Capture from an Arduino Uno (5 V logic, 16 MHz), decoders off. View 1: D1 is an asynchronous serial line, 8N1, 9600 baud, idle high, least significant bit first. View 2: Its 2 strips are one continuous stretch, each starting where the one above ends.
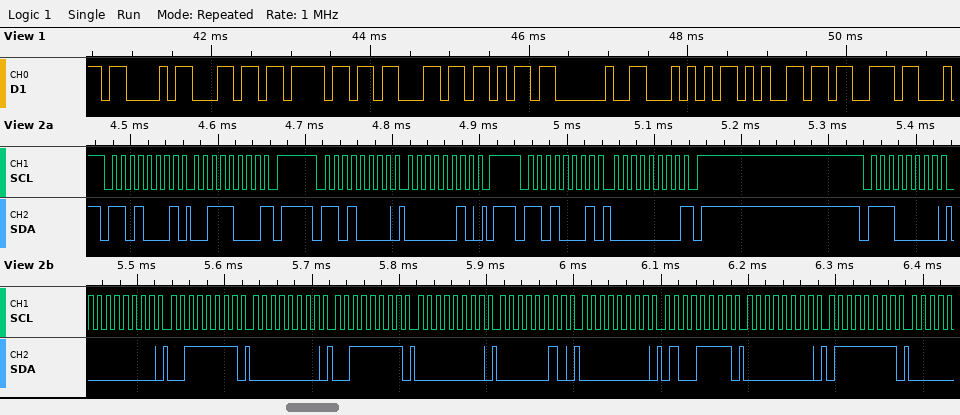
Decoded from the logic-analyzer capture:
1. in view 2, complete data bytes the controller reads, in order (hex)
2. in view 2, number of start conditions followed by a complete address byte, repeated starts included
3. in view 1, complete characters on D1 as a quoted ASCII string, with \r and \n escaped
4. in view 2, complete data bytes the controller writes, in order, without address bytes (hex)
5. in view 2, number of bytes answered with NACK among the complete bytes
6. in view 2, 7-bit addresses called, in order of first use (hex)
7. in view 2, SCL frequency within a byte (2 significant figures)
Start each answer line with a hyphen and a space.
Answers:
- 38 00
- 4
- "Clock Tes"
- 02 00 3F 00 3F 00 02 00 4F 00 7F
- 2
- 0x68 0x70
- 100 kHz
